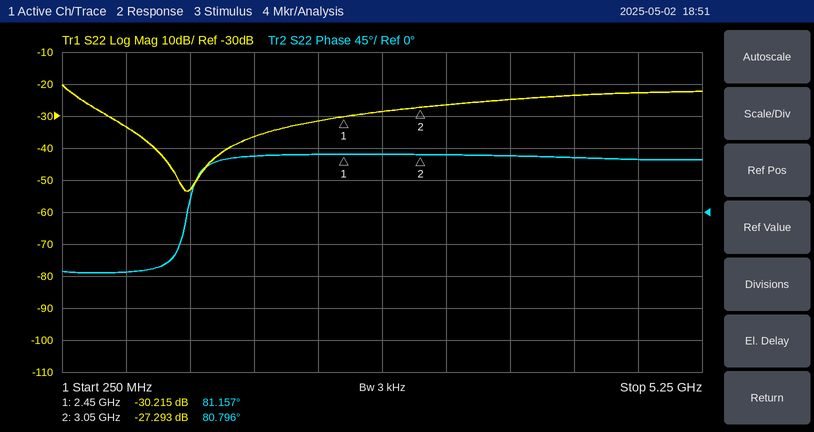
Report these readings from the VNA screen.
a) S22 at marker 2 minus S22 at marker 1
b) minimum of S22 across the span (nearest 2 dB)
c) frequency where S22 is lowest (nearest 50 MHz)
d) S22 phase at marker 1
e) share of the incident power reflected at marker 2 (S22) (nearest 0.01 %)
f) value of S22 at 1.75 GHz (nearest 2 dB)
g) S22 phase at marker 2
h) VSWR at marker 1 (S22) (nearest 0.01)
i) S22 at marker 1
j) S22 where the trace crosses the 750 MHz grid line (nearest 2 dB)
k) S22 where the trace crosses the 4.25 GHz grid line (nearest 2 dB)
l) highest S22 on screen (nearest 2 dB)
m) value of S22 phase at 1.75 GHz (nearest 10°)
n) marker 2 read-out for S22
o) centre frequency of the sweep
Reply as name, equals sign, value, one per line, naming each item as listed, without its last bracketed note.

S22 at marker 2 minus S22 at marker 1 = 2.922 dB
minimum of S22 across the span = -54 dB
frequency where S22 is lowest = 1.25 GHz
S22 phase at marker 1 = 81.157°
share of the incident power reflected at marker 2 (S22) = 0.19 %
value of S22 at 1.75 GHz = -36 dB
S22 phase at marker 2 = 80.796°
VSWR at marker 1 (S22) = 1.06
S22 at marker 1 = -30.215 dB
S22 where the trace crosses the 750 MHz grid line = -34 dB
S22 where the trace crosses the 4.25 GHz grid line = -24 dB
highest S22 on screen = -20 dB
value of S22 phase at 1.75 GHz = 80°
marker 2 read-out for S22 = -27.293 dB
centre frequency of the sweep = 2.75 GHz
